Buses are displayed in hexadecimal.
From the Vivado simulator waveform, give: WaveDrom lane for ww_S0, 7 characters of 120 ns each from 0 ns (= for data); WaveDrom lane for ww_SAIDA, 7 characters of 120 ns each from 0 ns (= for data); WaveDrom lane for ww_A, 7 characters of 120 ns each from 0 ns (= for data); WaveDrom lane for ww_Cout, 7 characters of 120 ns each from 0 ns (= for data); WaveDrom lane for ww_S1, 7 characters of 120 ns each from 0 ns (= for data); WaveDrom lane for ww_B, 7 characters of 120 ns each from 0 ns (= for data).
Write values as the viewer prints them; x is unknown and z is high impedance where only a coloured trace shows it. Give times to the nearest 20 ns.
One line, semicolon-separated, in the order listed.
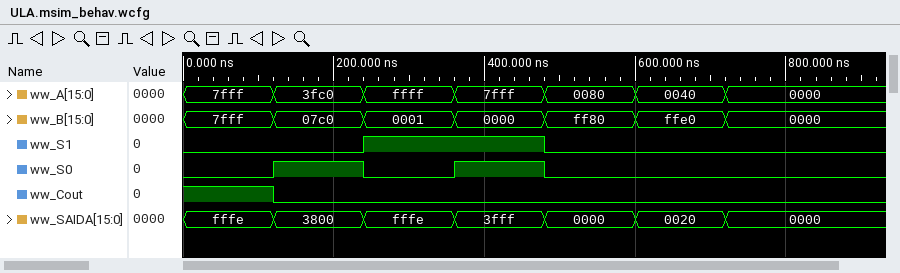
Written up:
{name: 'ww_S0', wave: '01010..'}; {name: 'ww_SAIDA', wave: '=======', data: 'fffe 3800 fffe 3fff 0000 0020 0000'}; {name: 'ww_A', wave: '=======', data: '7fff 3fc0 ffff 7fff 0080 0040 0000'}; {name: 'ww_Cout', wave: '10.....'}; {name: 'ww_S1', wave: '0.1.0..'}; {name: 'ww_B', wave: '=======', data: '7fff 07c0 0001 0000 ff80 ffe0 0000'}
